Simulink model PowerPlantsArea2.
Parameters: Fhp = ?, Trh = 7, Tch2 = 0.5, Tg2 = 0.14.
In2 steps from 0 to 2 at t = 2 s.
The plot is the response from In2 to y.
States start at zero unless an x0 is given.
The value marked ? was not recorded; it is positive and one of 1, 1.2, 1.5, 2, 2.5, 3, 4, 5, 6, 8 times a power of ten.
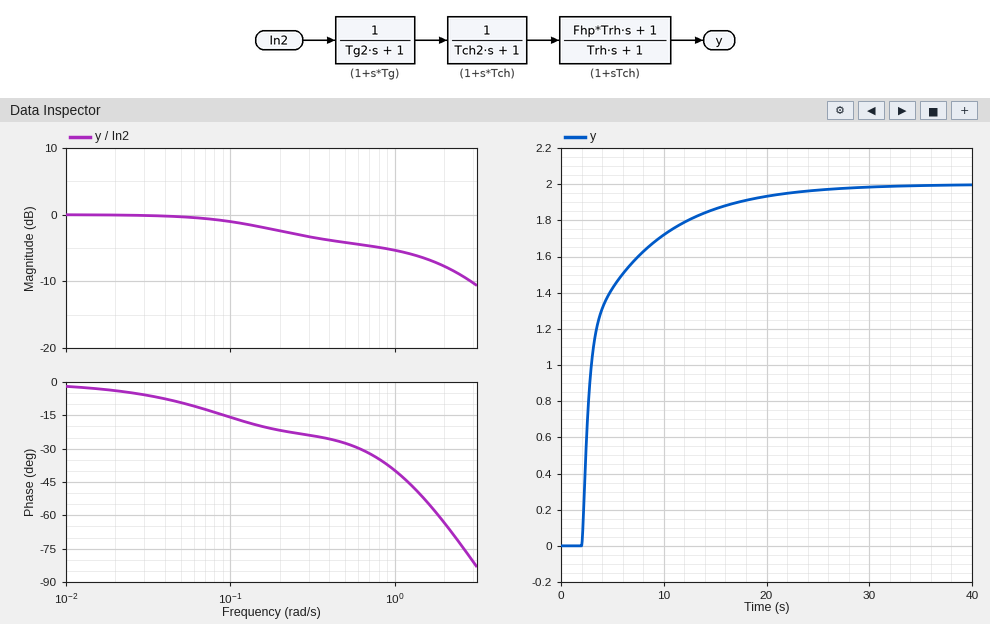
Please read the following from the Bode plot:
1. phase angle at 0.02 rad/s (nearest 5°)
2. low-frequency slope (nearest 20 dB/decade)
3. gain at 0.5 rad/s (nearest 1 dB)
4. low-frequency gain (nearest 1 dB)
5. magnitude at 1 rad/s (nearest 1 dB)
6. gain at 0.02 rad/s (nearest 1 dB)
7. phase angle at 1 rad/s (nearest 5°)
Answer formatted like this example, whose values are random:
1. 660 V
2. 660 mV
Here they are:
1. -5°
2. 0 dB/decade
3. -4 dB
4. 0 dB
5. -5 dB
6. 0 dB
7. -40°
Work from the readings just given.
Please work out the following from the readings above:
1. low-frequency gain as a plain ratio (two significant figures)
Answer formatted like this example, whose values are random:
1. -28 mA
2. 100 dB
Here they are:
1. 1.0
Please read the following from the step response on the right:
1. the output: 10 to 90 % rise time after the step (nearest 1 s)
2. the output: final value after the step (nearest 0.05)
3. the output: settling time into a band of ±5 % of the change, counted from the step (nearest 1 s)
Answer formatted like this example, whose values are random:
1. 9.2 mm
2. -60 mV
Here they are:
1. 10 s
2. 2.00
3. 15 s
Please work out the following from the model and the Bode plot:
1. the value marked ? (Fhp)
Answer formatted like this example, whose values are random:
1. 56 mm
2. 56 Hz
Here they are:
1. 0.6
